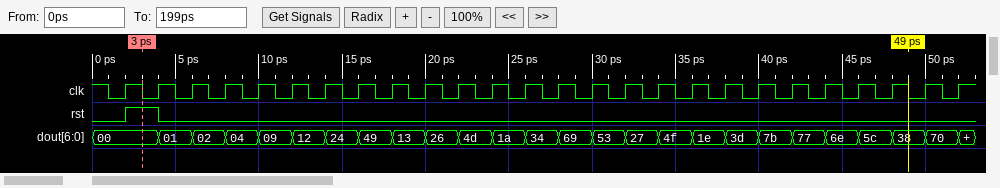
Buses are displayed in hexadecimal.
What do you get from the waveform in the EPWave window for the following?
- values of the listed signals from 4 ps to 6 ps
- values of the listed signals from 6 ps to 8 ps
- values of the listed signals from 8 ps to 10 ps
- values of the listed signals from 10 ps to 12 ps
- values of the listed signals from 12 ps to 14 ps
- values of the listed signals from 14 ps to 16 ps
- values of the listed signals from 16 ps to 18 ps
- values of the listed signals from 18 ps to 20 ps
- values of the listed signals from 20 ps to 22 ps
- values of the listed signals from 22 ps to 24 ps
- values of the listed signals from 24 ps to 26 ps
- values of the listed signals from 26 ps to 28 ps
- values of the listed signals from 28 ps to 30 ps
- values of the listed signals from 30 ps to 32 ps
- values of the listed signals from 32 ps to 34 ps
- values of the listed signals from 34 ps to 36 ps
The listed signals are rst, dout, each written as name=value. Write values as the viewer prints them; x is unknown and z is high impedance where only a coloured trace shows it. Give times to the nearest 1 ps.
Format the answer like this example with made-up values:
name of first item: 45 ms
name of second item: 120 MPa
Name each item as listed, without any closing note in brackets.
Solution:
values of the listed signals from 4 ps to 6 ps: rst=0, dout=01
values of the listed signals from 6 ps to 8 ps: rst=0, dout=02
values of the listed signals from 8 ps to 10 ps: rst=0, dout=04
values of the listed signals from 10 ps to 12 ps: rst=0, dout=09
values of the listed signals from 12 ps to 14 ps: rst=0, dout=12
values of the listed signals from 14 ps to 16 ps: rst=0, dout=24
values of the listed signals from 16 ps to 18 ps: rst=0, dout=49
values of the listed signals from 18 ps to 20 ps: rst=0, dout=13
values of the listed signals from 20 ps to 22 ps: rst=0, dout=26
values of the listed signals from 22 ps to 24 ps: rst=0, dout=4d
values of the listed signals from 24 ps to 26 ps: rst=0, dout=1a
values of the listed signals from 26 ps to 28 ps: rst=0, dout=34
values of the listed signals from 28 ps to 30 ps: rst=0, dout=69
values of the listed signals from 30 ps to 32 ps: rst=0, dout=53
values of the listed signals from 32 ps to 34 ps: rst=0, dout=27
values of the listed signals from 34 ps to 36 ps: rst=0, dout=4f
